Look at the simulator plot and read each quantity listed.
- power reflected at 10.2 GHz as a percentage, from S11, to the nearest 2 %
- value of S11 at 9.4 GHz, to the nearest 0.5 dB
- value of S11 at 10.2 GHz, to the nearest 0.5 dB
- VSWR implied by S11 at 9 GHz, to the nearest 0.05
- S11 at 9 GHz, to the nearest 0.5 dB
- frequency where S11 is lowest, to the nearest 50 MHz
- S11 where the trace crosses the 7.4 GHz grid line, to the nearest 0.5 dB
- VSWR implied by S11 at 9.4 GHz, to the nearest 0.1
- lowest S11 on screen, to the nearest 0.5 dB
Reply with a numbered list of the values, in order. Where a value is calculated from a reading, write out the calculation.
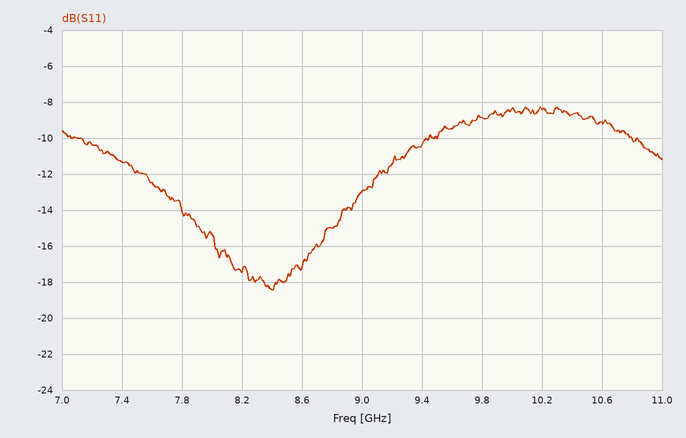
1. 10^(-8.5/10) ≈ 14 %
2. -10.5 dB
3. -8.5 dB
4. |Γ| = 10^(-13/20) = 0.2239; VSWR = (1 + 0.2239)/(1 − 0.2239) ≈ 1.58, so 1.60 to the nearest 0.05
5. -13.0 dB
6. 8.40 GHz
7. -11.5 dB
8. |Γ| = 10^(-10.5/20) = 0.2985; VSWR = (1 + 0.2985)/(1 − 0.2985) ≈ 1.9
9. -18.5 dB
